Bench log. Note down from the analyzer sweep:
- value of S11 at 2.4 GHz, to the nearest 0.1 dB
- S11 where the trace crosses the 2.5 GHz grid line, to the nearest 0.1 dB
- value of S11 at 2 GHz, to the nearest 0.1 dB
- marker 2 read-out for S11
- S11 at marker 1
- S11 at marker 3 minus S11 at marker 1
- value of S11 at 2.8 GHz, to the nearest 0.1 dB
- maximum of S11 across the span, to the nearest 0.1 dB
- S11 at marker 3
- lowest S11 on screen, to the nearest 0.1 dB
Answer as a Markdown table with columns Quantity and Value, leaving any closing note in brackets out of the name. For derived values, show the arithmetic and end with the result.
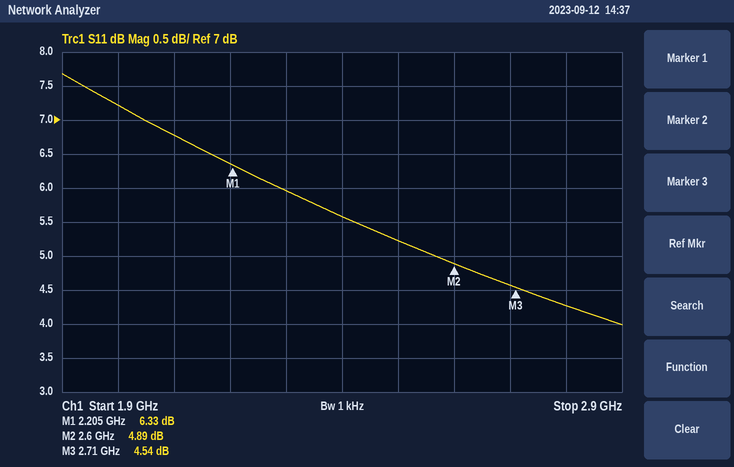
| Quantity | Value |
|---|---|
| value of S11 at 2.4 GHz, to the nearest 0.1 dB | 5.6 dB |
| S11 where the trace crosses the 2.5 GHz grid line, to the nearest 0.1 dB | 5.2 dB |
| value of S11 at 2 GHz, to the nearest 0.1 dB | 7.2 dB |
| marker 2 read-out for S11 | 4.89 dB |
| S11 at marker 1 | 6.33 dB |
| S11 at marker 3 minus S11 at marker 1 | 4.54 − (6.33) = -1.79 dB |
| value of S11 at 2.8 GHz, to the nearest 0.1 dB | 4.3 dB |
| maximum of S11 across the span, to the nearest 0.1 dB | 7.7 dB |
| S11 at marker 3 | 4.54 dB |
| lowest S11 on screen, to the nearest 0.1 dB | 4.0 dB |
